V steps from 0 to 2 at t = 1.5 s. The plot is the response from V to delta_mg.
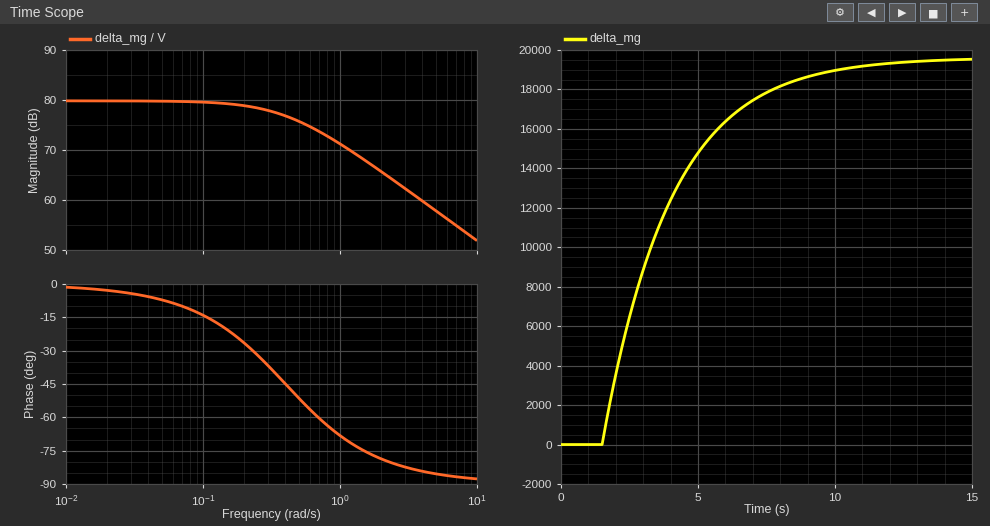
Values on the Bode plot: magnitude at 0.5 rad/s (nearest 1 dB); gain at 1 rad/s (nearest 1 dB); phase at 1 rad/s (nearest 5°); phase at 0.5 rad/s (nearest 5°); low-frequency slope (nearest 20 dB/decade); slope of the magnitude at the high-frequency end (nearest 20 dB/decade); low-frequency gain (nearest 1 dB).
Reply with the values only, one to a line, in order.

76 dB
71 dB
-70°
-50°
0 dB/decade
-20 dB/decade
80 dB
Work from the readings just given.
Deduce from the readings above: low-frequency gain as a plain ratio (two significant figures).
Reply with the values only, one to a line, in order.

10000
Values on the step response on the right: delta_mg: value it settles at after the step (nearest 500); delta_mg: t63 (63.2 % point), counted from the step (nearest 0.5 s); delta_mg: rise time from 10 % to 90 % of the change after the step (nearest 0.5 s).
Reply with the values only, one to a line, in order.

19500
2.5 s
5.5 s
